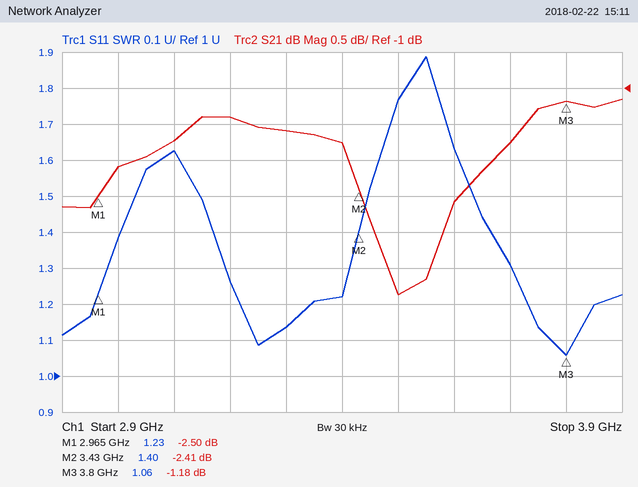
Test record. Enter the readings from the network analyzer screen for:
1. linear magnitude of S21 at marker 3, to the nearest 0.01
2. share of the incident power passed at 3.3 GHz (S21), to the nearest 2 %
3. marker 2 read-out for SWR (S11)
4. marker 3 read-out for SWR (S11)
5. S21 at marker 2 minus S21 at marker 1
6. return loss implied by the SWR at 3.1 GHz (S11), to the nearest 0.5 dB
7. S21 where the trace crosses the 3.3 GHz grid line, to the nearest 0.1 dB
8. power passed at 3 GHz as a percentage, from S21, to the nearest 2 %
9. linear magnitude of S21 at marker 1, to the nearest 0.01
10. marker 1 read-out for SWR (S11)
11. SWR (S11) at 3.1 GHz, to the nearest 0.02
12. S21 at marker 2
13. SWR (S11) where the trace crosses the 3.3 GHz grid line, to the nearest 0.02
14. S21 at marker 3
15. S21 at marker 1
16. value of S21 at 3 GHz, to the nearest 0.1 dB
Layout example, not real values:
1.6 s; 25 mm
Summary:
0.87; 70 %; 1.40; 1.06; 0.09 dB; 12.5 dB; -1.6 dB; 62 %; 0.75; 1.23; 1.62; -2.41 dB; 1.14; -1.18 dB; -2.50 dB; -2.1 dB
